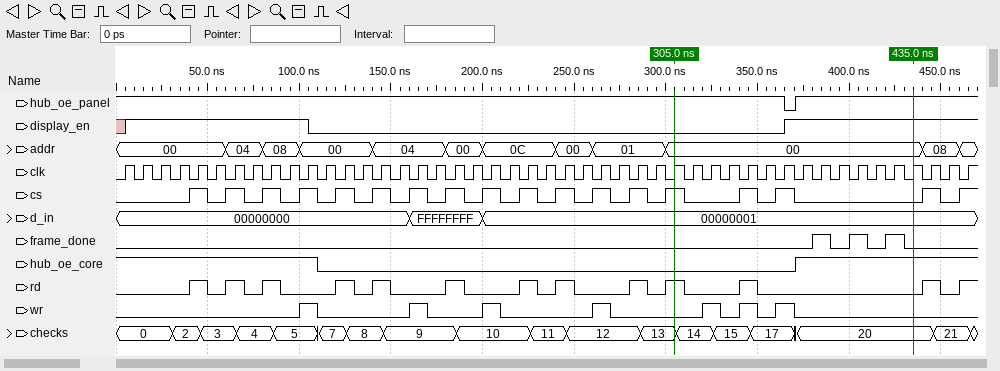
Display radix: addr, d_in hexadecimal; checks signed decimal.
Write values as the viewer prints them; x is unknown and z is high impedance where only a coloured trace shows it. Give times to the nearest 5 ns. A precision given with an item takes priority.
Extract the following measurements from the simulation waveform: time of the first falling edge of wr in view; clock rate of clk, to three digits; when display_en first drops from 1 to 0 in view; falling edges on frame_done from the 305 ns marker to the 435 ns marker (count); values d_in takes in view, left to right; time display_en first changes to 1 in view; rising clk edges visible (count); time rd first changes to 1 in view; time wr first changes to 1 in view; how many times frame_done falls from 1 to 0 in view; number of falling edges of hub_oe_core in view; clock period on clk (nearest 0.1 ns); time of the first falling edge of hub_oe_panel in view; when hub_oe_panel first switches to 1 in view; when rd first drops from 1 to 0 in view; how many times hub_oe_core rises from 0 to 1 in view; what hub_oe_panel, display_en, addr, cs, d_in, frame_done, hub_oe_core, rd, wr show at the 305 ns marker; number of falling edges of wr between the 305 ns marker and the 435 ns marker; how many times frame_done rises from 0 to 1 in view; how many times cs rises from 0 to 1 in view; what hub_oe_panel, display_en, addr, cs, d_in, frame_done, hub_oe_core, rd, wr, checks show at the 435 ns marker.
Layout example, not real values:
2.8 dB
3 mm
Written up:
110 ns
100 MHz
105 ns
3
00000000, FFFFFFFF, 00000001
5 ns
47
40 ns
100 ns
3
1
10 ns
365 ns
370 ns
50 ns
1
hub_oe_panel=1, display_en=0, addr=00, cs=1, d_in=00000001, frame_done=0, hub_oe_core=0, rd=1, wr=0
3
3
18
hub_oe_panel=1, display_en=1, addr=00, cs=0, d_in=00000001, frame_done=0, hub_oe_core=1, rd=0, wr=0, checks=20
